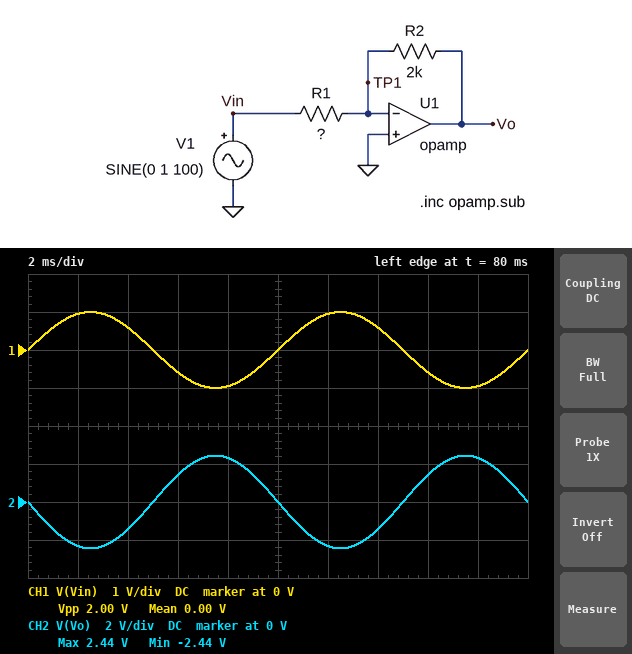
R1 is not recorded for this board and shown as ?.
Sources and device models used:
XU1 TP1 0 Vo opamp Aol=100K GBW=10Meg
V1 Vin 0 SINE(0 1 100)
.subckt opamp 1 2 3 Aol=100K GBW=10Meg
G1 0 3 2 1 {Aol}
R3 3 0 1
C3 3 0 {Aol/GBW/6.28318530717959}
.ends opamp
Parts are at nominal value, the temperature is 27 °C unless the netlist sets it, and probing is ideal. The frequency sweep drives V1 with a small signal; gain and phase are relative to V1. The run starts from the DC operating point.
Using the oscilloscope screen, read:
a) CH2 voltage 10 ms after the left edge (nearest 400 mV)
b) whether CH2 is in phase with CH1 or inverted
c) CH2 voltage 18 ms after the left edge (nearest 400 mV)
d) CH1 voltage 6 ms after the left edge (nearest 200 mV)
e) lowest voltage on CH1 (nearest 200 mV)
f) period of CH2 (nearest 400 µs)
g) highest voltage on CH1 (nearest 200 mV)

0 V
inverted
2.4 V
-600 mV
-1.0 V
10.0 ms
1.0 V
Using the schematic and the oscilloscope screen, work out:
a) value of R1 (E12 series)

820 Ω
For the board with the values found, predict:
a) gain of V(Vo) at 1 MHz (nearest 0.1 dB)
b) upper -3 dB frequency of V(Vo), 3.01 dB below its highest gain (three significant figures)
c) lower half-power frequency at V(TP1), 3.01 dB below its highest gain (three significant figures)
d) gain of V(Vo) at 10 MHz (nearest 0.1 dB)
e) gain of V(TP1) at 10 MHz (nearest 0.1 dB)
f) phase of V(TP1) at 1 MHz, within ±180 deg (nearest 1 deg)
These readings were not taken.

7.3 dB
2.91 MHz
2.91 MHz
-3.3 dB
-3.3 dB
71 deg
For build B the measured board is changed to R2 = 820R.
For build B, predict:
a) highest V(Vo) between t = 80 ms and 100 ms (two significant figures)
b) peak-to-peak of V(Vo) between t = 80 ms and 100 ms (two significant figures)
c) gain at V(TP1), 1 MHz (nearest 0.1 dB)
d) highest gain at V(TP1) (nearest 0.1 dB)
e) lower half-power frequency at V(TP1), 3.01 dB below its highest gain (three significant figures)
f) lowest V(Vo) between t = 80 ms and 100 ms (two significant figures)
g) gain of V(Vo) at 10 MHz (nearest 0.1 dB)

1.0 V
2.0 V
-20.2 dB
-6.0 dB
5.00 MHz
-1.0 V
-7.0 dB
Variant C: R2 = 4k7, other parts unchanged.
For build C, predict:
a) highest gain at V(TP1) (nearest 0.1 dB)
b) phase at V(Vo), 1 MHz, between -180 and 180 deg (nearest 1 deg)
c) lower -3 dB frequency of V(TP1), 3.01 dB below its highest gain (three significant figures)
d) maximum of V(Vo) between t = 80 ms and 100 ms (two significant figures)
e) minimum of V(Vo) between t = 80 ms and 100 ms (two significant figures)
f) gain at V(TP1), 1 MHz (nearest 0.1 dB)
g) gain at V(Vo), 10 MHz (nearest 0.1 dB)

-1.4 dB
146 deg
1.49 MHz
5.7 V
-5.7 V
-6.5 dB
-1.5 dB
